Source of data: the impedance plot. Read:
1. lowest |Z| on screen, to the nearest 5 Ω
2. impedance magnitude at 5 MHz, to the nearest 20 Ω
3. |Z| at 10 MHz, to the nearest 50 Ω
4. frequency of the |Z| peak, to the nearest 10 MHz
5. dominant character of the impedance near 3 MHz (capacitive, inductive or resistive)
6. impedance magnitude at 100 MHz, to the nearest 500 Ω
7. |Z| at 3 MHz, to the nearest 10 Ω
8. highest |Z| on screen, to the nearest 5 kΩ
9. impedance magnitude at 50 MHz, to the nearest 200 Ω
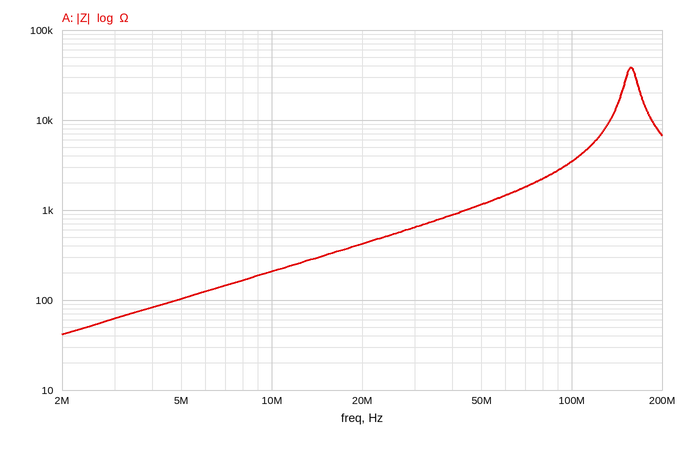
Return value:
40 Ω
100 Ω
200 Ω
160 MHz
inductive
3.5 kΩ
60 Ω
40 kΩ
1.2 kΩ
